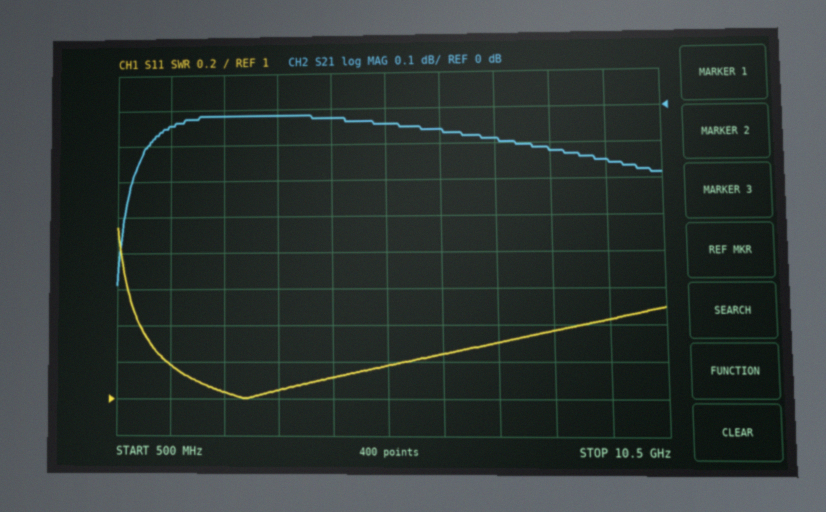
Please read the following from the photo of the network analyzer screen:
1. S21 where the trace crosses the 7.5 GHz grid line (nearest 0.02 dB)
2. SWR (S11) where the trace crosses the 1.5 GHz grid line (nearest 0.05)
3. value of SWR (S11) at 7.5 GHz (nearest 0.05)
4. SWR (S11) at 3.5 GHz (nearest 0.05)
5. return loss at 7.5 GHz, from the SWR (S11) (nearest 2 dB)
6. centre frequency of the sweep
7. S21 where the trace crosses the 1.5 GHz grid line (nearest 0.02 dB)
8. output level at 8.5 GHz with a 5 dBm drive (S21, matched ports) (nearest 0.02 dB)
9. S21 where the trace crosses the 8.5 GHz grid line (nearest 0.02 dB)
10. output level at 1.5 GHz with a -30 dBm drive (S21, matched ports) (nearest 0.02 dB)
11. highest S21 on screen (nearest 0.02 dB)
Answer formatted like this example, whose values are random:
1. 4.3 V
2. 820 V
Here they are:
1. -0.08 dB
2. 1.20
3. 1.30
4. 1.05
5. 18 dB
6. 5.5 GHz
7. -0.04 dB
8. 4.88 dBm
9. -0.12 dB
10. -30.04 dBm
11. -0.02 dB
